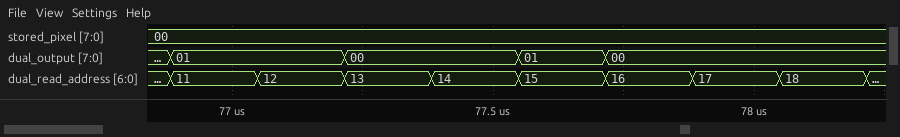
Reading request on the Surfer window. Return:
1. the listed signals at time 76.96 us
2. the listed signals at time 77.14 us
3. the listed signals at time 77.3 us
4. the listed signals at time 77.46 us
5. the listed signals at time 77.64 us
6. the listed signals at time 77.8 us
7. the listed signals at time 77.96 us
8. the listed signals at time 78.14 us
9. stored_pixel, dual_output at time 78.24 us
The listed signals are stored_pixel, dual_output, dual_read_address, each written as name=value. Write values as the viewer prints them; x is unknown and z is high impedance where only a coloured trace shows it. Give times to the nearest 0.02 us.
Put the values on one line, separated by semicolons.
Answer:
stored_pixel=00, dual_output=01, dual_read_address=11; stored_pixel=00, dual_output=01, dual_read_address=12; stored_pixel=00, dual_output=00, dual_read_address=13; stored_pixel=00, dual_output=00, dual_read_address=14; stored_pixel=00, dual_output=01, dual_read_address=15; stored_pixel=00, dual_output=00, dual_read_address=16; stored_pixel=00, dual_output=00, dual_read_address=17; stored_pixel=00, dual_output=00, dual_read_address=18; stored_pixel=00, dual_output=00
